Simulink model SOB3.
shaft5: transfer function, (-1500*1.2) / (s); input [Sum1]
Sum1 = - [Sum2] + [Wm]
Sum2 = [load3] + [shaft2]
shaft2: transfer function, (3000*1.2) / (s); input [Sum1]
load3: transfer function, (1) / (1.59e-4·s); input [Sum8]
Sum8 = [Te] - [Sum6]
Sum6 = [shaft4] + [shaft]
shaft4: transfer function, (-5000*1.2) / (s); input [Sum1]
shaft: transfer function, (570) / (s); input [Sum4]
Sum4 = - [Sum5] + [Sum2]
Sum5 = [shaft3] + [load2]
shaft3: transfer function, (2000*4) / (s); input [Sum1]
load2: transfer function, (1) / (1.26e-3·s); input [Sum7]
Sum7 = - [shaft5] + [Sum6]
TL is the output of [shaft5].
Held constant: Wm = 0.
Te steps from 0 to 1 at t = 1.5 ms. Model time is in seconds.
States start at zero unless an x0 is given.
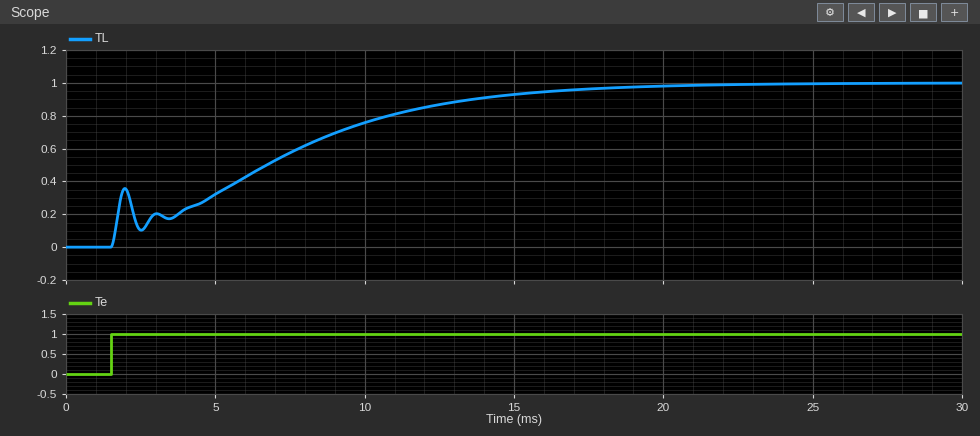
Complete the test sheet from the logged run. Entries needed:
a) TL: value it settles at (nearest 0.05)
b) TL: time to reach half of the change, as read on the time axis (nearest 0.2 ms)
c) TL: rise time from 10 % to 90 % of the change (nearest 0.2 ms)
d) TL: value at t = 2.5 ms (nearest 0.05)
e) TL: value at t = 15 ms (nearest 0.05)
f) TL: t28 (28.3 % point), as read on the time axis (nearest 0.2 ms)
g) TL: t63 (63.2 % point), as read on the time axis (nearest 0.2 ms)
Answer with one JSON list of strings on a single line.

["1.00", "6.8 ms", "12.0 ms", "0.10", "0.95", "1.8 ms", "8.2 ms"]
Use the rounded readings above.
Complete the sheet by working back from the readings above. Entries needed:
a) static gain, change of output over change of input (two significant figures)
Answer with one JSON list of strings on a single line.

["1.0"]
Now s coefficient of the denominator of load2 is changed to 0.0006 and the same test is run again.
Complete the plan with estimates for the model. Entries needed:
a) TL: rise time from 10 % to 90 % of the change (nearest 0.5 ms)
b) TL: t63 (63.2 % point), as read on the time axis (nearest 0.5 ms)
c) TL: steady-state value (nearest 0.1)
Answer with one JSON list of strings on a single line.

["6.0 ms", "5.5 ms", "1.0"]
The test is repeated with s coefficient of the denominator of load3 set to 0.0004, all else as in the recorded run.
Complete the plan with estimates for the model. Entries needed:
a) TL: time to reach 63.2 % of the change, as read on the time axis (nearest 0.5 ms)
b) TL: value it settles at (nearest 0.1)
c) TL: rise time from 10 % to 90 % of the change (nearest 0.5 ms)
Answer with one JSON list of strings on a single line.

["8.5 ms", "1.0", "13.0 ms"]
